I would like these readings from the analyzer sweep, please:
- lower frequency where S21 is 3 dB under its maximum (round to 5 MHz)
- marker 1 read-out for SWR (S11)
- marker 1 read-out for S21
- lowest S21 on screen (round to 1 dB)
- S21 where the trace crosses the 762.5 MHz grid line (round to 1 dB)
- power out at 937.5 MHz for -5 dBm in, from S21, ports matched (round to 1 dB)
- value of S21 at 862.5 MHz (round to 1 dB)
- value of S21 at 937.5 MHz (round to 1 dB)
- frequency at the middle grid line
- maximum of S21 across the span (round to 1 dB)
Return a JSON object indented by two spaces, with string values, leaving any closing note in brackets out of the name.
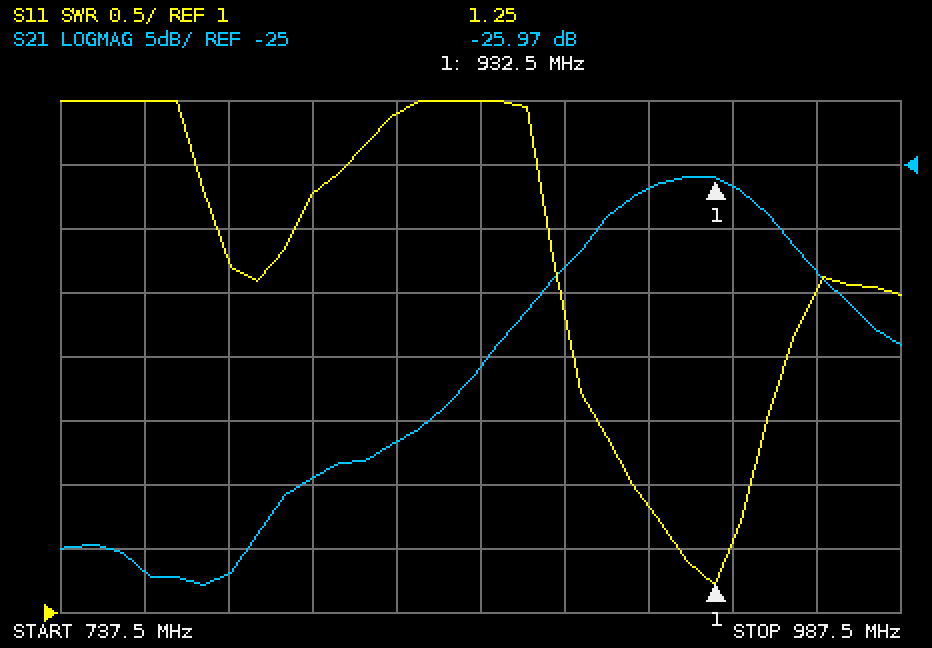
{
  "lower frequency where S21 is 3 dB under its maximum": "900 MHz",
  "marker 1 read-out for SWR": "1.25",
  "marker 1 read-out for S21": "-25.97 dB",
  "lowest S21 on screen": "-58 dB",
  "S21 where the trace crosses the 762.5 MHz grid line": "-57 dB",
  "power out at 937.5 MHz for -5 dBm in, from S21, ports matched": "-32 dBm",
  "value of S21 at 862.5 MHz": "-41 dB",
  "value of S21 at 937.5 MHz": "-27 dB",
  "frequency at the middle grid line": "862.5 MHz",
  "maximum of S21 across the span": "-26 dB"
}
